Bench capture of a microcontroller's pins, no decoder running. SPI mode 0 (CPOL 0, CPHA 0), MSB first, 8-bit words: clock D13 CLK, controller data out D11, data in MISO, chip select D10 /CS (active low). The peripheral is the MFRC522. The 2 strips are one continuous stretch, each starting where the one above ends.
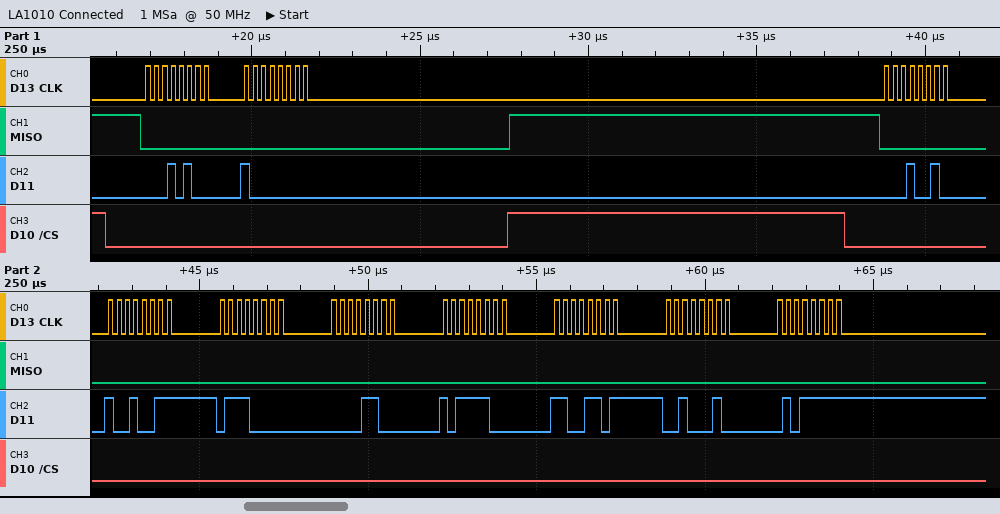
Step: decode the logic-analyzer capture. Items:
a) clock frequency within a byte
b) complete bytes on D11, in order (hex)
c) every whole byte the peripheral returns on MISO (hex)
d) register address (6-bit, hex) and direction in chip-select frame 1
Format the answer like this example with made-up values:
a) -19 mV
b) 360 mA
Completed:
a) 4 MHz
b) 14 80 12 93 70 0C BC CD 22 5F
c) 00 00 00 00 00 00 00 00 00 00
d) 0x0A write
